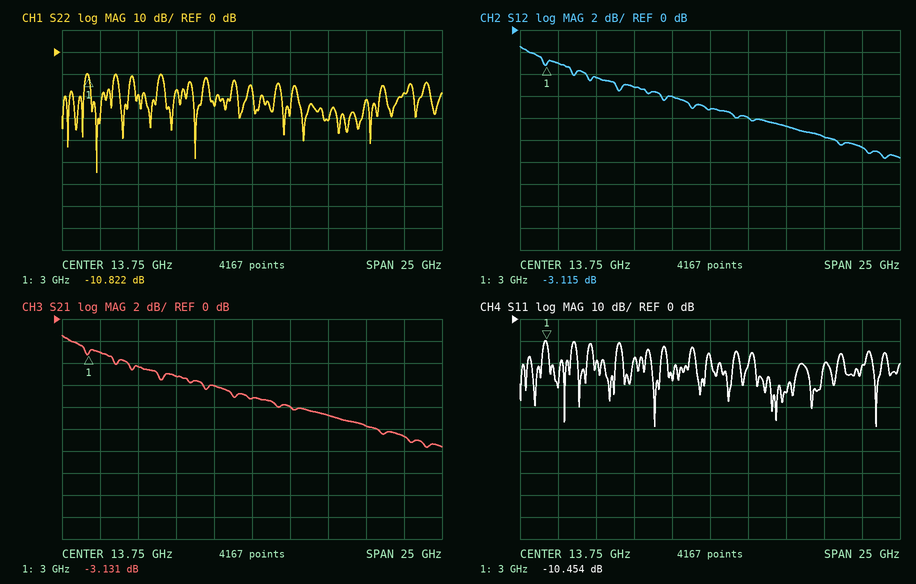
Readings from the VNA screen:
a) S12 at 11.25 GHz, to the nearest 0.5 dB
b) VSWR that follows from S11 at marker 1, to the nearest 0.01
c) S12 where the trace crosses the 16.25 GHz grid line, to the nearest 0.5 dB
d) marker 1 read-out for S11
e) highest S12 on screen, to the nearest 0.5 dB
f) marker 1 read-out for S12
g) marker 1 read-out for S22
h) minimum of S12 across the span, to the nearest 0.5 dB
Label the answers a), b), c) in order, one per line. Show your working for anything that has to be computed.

a) -6.0 dB
b) (1 + 0.3001)/(1 − 0.3001) ≈ 1.86
c) -8.0 dB
d) -10.454 dB
e) -1.5 dB
f) -3.115 dB
g) -10.822 dB
h) -11.5 dB
